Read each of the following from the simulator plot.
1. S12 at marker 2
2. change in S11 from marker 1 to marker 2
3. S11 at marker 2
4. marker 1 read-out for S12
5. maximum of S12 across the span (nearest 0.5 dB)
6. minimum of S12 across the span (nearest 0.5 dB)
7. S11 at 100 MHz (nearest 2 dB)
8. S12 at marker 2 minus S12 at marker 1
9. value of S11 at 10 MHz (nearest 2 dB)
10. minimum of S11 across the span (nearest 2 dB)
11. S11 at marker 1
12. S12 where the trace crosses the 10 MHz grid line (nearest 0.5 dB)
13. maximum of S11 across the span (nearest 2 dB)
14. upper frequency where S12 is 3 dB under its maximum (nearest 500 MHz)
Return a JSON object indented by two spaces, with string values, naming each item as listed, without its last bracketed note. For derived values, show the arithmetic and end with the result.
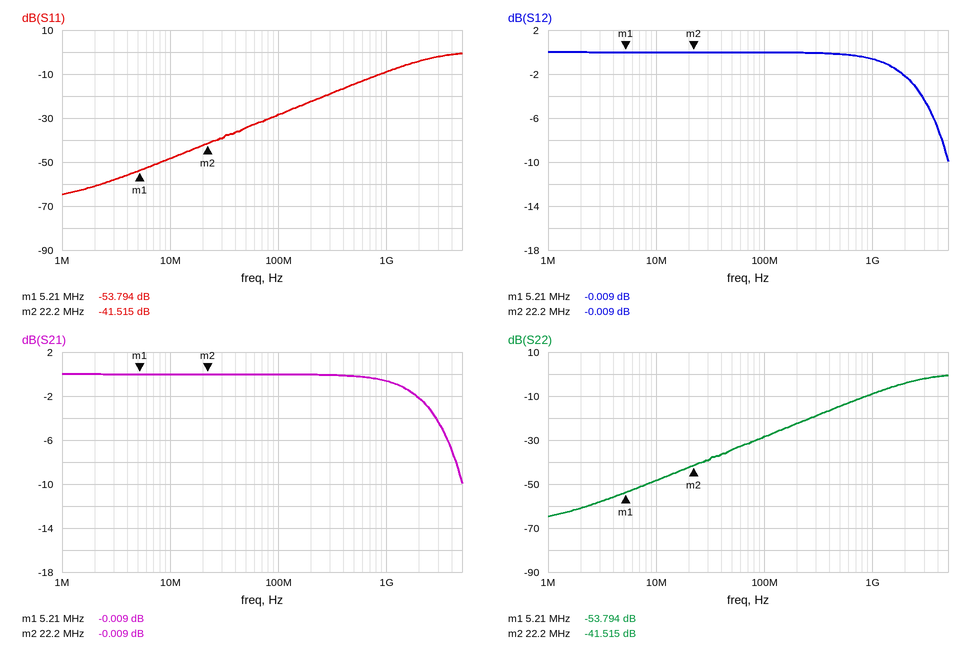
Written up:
{
  "S12 at marker 2": "-0.009 dB",
  "change in S11 from marker 1 to marker 2": "-41.515 − (-53.794) = 12.279 dB",
  "S11 at marker 2": "-41.515 dB",
  "marker 1 read-out for S12": "-0.009 dB",
  "maximum of S12 across the span": "0.0 dB",
  "minimum of S12 across the span": "-10.0 dB",
  "S11 at 100 MHz": "-28 dB",
  "S12 at marker 2 minus S12 at marker 1": "-0.009 − (-0.009) = 0.000 dB",
  "value of S11 at 10 MHz": "-48 dB",
  "minimum of S11 across the span": "-64 dB",
  "S11 at marker 1": "-53.794 dB",
  "S12 where the trace crosses the 10 MHz grid line": "0.0 dB",
  "maximum of S11 across the span": "0 dB",
  "upper frequency where S12 is 3 dB under its maximum": "2.5 GHz"
}
